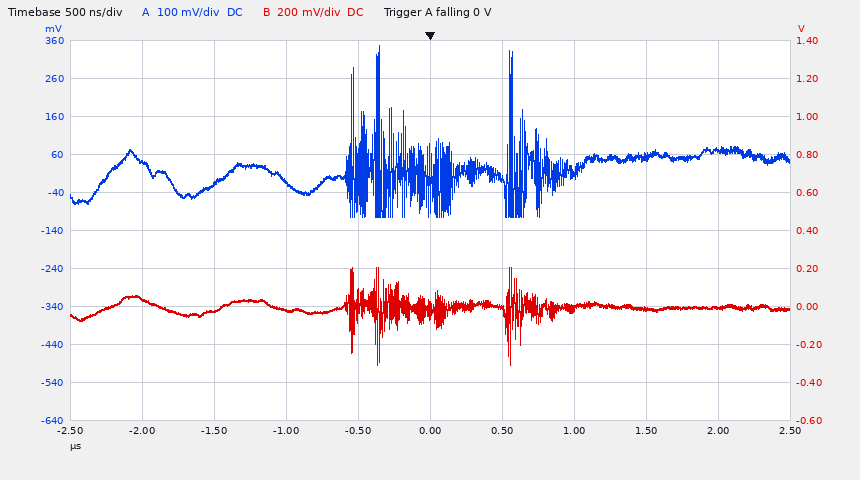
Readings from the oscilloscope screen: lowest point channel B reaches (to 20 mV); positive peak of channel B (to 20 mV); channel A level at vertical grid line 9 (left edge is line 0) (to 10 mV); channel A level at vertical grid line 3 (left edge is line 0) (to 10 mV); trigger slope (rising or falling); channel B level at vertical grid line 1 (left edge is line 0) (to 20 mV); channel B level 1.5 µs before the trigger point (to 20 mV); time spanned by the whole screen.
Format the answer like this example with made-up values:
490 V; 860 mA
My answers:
-300 mV; 200 mV; 70 mV; -10 mV; falling; 40 mV; -20 mV; 5 µs
